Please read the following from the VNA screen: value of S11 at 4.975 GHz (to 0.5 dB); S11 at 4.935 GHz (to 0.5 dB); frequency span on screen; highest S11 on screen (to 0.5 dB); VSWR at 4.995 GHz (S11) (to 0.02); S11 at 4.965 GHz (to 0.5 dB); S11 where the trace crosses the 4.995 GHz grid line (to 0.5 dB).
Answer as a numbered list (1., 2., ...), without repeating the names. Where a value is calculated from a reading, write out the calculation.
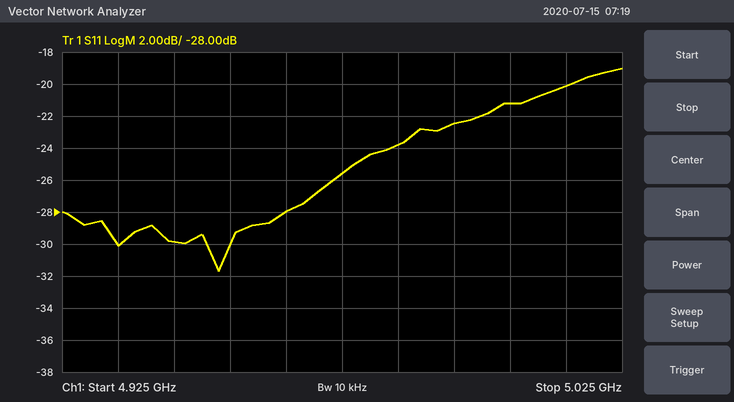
1. -25.5 dB
2. -30.0 dB
3. 100 MHz
4. -19.0 dB
5. |Γ| = 10^(-22.5/20) = 0.0750; VSWR = (1 + 0.0750)/(1 − 0.0750) ≈ 1.16
6. -28.0 dB
7. -22.5 dB
